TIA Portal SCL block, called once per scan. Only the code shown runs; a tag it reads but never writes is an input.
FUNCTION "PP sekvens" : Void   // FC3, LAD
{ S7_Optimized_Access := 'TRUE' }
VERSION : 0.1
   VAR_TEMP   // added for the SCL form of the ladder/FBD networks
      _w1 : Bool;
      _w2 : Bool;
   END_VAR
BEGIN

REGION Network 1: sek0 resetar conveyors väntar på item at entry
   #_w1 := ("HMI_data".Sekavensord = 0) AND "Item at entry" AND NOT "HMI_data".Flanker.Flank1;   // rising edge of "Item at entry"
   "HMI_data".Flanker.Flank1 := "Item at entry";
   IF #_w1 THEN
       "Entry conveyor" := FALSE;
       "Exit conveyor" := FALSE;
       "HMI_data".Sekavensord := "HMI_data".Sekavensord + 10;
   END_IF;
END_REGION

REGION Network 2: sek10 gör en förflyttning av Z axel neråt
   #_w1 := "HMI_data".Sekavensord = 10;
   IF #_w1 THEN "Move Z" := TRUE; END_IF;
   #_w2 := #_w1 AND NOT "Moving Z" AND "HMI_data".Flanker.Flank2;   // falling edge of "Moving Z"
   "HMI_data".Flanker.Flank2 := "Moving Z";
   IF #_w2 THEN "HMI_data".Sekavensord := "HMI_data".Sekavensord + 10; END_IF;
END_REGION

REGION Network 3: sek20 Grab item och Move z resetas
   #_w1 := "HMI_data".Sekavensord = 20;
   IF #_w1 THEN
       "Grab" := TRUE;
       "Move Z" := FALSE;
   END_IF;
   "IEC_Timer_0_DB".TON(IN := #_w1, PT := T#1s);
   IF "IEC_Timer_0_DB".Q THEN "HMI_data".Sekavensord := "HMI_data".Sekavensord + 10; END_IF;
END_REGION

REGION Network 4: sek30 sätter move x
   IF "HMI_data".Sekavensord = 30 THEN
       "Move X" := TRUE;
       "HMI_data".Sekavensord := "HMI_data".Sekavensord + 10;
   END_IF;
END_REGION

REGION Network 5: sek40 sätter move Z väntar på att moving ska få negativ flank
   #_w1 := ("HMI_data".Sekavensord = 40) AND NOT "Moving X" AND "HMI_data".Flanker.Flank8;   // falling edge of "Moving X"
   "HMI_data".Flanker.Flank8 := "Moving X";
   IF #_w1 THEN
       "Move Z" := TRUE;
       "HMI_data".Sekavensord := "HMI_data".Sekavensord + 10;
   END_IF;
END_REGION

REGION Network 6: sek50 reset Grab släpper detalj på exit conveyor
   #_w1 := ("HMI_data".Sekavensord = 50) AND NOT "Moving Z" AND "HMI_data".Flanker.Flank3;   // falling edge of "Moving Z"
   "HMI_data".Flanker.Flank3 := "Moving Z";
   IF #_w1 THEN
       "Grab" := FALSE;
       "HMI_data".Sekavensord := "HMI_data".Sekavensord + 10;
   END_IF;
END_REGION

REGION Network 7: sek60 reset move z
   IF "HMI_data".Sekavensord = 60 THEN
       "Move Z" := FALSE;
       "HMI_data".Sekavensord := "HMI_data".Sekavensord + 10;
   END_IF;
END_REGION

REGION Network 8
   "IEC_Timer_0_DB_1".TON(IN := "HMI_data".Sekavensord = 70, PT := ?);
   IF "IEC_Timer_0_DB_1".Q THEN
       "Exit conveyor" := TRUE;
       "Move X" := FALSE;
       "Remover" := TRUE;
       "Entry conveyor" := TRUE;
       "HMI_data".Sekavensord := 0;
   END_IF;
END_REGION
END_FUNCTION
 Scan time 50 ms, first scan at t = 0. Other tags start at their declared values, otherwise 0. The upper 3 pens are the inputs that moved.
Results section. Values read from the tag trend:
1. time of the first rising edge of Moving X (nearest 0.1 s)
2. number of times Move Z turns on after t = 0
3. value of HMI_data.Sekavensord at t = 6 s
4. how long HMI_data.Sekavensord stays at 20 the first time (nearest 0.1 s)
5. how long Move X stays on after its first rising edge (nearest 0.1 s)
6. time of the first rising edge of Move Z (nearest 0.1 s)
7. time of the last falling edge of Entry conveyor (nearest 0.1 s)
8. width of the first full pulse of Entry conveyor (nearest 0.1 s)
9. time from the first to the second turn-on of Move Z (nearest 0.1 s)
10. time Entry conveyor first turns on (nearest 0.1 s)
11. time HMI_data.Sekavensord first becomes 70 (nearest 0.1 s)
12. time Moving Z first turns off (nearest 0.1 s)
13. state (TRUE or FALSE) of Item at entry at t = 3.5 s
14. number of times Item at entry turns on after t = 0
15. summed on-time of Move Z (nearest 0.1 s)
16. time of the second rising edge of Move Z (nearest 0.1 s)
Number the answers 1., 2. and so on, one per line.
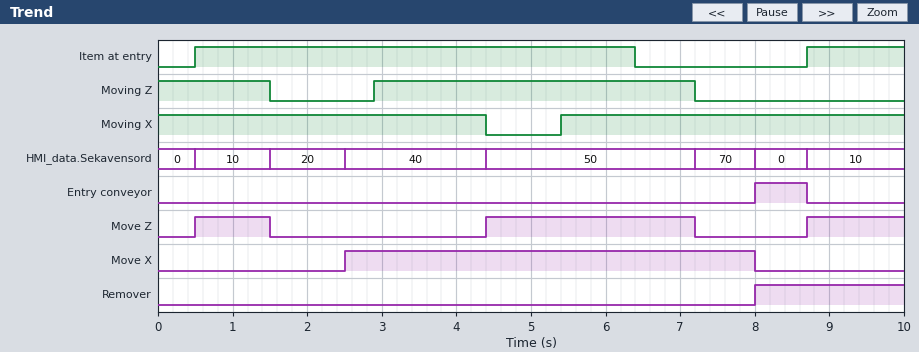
1. 5.4 s
2. 3
3. 50
4. 1.0 s
5. 5.5 s
6. 0.5 s
7. 8.7 s
8. 0.7 s
9. 3.9 s
10. 8.0 s
11. 7.2 s
12. 1.5 s
13. TRUE
14. 2
15. 5.1 s
16. 4.4 s
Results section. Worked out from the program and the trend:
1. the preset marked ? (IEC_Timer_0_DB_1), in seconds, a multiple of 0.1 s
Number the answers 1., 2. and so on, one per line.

1. 0.8 s
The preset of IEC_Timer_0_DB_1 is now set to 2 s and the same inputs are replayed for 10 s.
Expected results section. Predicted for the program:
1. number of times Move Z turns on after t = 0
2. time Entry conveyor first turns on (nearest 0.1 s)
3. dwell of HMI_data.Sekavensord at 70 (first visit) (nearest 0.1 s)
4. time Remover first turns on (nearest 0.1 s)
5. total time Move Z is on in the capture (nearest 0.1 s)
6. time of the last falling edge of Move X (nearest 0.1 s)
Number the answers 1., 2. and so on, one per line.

1. 2
2. 9.2 s
3. 2.0 s
4. 9.2 s
5. 3.8 s
6. 9.2 s
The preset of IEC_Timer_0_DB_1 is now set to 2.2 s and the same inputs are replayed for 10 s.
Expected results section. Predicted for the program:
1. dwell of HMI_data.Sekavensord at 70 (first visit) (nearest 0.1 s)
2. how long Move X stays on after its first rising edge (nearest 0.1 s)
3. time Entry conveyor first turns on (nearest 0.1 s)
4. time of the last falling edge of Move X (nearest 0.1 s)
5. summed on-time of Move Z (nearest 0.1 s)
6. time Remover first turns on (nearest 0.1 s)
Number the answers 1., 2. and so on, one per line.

1. 2.2 s
2. 6.9 s
3. 9.4 s
4. 9.4 s
5. 3.8 s
6. 9.4 s
